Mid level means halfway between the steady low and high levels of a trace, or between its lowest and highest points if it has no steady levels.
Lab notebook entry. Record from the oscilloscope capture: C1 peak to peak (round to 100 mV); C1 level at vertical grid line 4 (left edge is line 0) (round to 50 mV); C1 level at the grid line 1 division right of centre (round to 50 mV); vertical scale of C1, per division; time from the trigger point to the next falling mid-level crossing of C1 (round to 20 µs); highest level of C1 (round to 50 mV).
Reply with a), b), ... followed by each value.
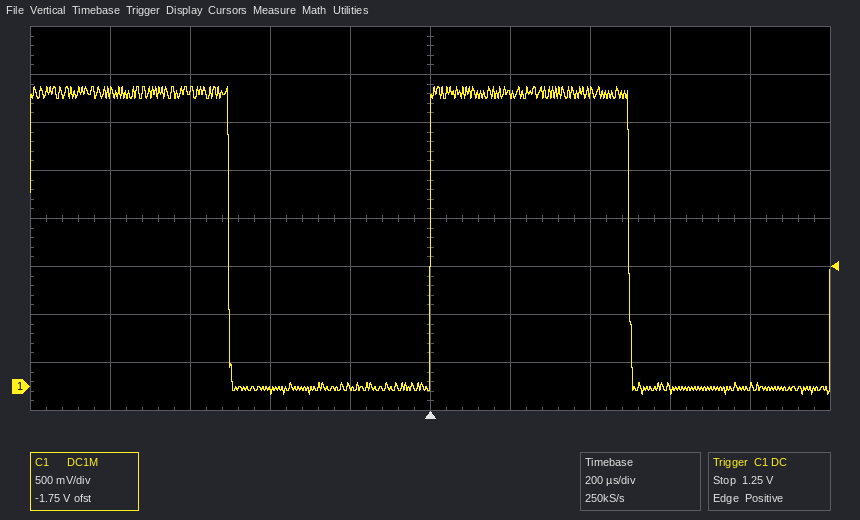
a) 3.20 V
b) 0 mV
c) 3.05 V
d) 500 mV
e) 500 µs
f) 3.10 V
